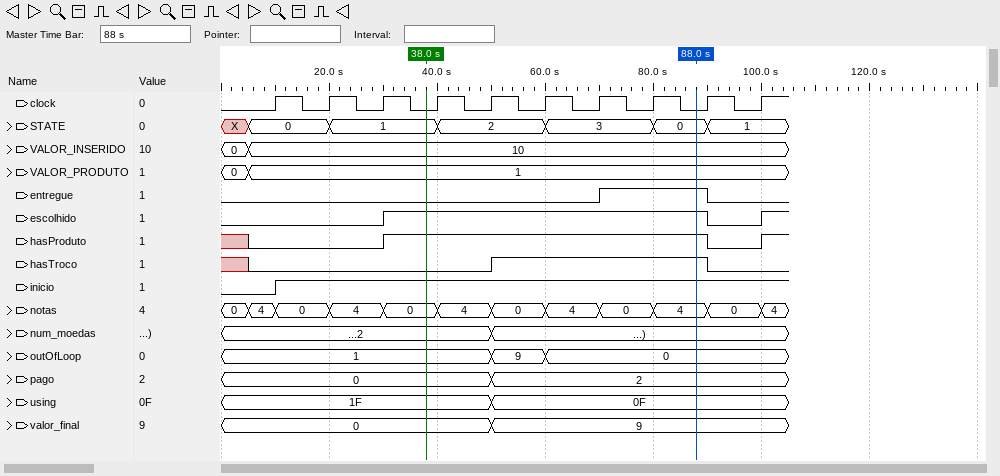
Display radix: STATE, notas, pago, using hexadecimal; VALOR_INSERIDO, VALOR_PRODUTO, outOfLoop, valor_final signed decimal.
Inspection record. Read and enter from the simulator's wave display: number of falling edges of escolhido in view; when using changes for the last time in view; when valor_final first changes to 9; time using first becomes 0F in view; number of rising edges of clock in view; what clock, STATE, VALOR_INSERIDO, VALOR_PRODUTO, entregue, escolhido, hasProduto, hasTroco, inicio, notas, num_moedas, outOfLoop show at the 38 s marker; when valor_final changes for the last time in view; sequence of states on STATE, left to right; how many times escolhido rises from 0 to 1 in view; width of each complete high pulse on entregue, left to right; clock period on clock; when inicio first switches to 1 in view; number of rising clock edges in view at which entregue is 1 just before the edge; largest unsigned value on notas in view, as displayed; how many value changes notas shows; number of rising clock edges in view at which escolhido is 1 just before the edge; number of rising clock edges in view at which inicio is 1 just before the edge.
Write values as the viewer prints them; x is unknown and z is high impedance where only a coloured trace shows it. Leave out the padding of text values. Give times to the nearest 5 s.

1
50 s
50 s
50 s
10
clock=0, STATE=1, VALOR_INSERIDO=10, VALOR_PRODUTO=1, entregue=0, escolhido=1, hasProduto=1, hasTroco=0, inicio=1, notas=0, num_moedas=2, outOfLoop=1
50 s
X, 0, 1, 2, 3, 0, 1
2
20 s
10 s
10 s
2
4
11
6
9
